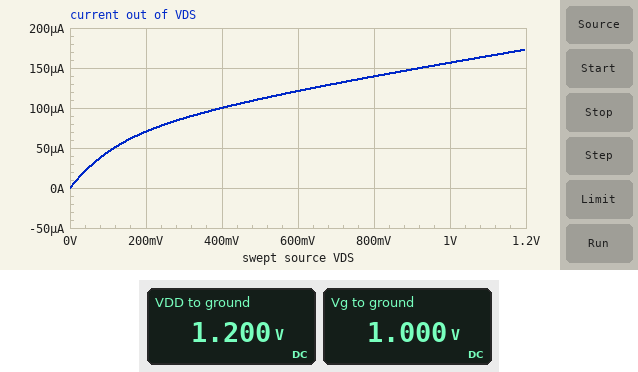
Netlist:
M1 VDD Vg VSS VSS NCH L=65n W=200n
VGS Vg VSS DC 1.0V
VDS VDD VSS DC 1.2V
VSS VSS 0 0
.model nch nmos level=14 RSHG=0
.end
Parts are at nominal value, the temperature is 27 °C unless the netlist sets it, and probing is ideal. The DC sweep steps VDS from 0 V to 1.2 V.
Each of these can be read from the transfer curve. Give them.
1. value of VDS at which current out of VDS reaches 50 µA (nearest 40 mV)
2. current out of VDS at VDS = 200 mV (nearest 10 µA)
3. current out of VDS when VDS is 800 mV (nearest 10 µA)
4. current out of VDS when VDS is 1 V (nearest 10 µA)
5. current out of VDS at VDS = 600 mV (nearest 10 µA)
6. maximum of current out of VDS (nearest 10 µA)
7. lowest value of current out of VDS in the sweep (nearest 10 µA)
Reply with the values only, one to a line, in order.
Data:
120 mV
70 µA
140 µA
160 µA
120 µA
170 µA
0 A
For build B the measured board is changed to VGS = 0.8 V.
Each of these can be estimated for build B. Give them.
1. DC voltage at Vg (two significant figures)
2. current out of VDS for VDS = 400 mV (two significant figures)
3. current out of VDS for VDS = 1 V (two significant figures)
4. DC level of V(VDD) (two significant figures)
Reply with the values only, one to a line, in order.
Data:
800 mV
72 µA
120 µA
1.2 V
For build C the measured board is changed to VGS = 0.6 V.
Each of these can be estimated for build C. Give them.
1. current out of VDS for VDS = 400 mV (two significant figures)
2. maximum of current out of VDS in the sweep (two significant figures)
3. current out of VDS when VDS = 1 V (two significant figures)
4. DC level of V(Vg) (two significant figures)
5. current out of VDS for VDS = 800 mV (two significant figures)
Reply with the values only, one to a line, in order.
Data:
43 µA
95 µA
82 µA
600 mV
69 µA
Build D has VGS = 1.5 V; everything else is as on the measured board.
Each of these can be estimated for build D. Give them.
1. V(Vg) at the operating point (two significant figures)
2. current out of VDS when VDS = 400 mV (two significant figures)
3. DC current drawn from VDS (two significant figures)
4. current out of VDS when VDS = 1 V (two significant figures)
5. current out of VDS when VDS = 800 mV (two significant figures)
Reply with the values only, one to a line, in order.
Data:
1.5 V
170 µA
270 µA
250 µA
230 µA
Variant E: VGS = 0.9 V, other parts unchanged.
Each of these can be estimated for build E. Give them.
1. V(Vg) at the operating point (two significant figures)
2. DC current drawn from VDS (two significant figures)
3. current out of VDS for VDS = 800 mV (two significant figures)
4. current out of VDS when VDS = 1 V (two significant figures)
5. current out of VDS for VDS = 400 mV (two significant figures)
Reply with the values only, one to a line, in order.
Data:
900 mV
150 µA
120 µA
140 µA
86 µA
